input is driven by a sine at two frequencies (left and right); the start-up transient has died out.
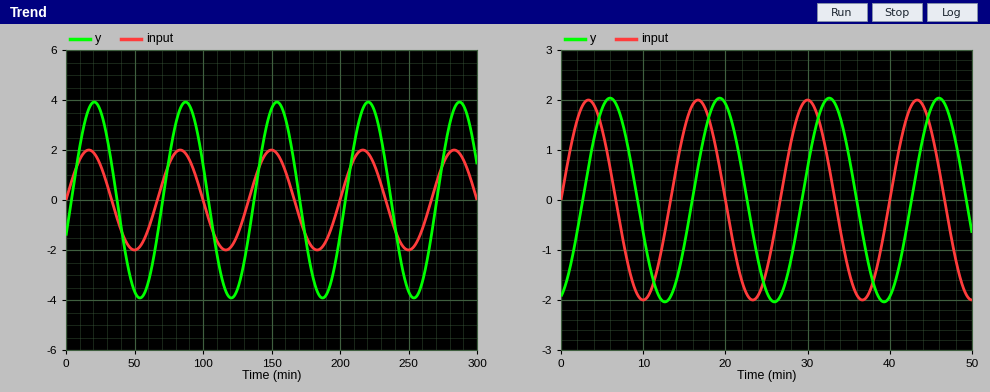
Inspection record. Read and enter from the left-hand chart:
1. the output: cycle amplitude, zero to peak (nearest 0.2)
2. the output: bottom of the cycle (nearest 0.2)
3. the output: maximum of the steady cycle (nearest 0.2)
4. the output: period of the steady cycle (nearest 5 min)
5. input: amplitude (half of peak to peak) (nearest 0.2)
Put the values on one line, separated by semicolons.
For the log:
4.0; -4.0; 4.0; 65 min; 2.0
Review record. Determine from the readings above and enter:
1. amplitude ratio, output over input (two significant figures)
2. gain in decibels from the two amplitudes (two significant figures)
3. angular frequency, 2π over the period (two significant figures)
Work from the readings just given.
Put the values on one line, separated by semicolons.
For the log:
2.0; 6.0 dB; 0.097 rad/min
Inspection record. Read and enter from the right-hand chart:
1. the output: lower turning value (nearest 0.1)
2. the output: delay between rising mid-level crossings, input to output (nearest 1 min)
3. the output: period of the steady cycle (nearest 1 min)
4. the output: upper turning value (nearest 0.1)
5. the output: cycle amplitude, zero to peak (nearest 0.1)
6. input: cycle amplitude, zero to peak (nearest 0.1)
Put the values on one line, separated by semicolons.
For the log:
-2.0; 3 min; 13 min; 2.0; 2.0; 2.0
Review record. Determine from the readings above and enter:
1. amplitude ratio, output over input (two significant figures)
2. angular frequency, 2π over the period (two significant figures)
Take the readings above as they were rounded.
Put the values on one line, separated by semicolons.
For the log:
1.0; 0.48 rad/min
